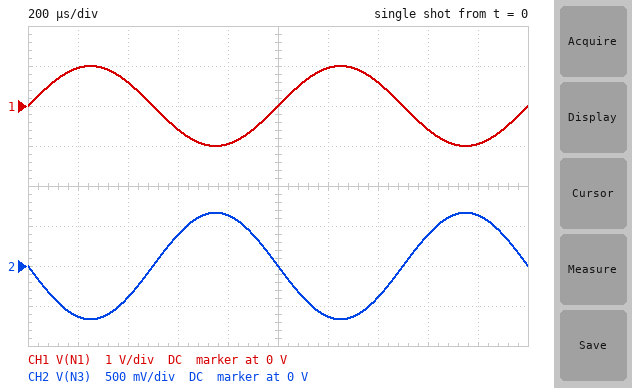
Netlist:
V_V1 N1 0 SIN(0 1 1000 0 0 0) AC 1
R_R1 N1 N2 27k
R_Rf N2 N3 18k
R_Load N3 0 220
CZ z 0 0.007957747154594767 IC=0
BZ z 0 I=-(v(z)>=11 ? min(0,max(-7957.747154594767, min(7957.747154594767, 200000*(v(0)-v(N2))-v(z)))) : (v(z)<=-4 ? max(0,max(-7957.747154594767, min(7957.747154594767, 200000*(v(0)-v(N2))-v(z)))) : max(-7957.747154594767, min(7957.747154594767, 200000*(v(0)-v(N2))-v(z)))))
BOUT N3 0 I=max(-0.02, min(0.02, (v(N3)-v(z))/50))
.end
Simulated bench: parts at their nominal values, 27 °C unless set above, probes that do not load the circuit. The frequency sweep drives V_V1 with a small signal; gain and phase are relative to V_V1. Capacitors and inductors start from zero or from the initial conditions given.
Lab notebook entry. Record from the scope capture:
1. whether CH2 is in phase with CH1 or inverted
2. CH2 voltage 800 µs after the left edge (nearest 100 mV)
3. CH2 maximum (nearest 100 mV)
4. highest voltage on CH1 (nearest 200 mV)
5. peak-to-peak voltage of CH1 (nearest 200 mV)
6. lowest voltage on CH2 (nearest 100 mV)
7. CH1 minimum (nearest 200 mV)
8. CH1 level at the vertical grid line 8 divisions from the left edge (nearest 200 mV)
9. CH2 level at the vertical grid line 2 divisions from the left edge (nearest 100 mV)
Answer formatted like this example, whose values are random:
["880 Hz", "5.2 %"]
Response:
["inverted", "600 mV", "700 mV", "1.0 V", "2.0 V", "-700 mV", "-1.0 V", "-600 mV", "-400 mV"]
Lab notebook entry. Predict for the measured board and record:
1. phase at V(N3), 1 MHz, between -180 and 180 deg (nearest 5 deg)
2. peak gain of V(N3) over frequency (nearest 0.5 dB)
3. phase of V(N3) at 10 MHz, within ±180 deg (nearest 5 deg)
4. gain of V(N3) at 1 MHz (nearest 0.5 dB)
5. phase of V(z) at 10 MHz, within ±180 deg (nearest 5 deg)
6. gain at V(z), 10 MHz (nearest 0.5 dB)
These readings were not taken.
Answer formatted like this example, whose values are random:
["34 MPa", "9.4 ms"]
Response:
["155 deg", "-3.5 dB", "100 deg", "-4.5 dB", "100 deg", "-16.0 dB"]
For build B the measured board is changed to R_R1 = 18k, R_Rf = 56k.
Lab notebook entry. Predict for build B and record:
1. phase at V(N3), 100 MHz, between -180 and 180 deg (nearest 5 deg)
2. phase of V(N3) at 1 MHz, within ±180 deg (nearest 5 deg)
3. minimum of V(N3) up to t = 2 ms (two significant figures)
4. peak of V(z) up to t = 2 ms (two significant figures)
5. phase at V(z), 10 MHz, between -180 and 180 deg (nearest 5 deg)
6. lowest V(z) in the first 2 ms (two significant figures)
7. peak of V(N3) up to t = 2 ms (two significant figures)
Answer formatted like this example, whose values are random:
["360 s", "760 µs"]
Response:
["90 deg", "130 deg", "-3.1 V", "3.8 V", "95 deg", "-3.8 V", "3.1 V"]
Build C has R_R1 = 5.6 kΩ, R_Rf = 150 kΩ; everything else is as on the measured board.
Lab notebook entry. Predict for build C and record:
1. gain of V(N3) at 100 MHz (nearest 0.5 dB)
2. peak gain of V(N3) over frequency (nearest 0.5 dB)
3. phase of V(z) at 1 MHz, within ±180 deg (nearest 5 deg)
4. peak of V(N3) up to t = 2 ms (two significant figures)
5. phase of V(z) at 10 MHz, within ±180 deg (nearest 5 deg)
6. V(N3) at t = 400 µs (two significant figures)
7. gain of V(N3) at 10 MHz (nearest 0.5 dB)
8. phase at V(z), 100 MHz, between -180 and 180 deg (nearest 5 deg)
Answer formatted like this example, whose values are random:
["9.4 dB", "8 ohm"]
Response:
["-30.0 dB", "28.5 dB", "95 deg", "4.4 V", "90 deg", "-3.3 V", "-10.0 dB", "90 deg"]
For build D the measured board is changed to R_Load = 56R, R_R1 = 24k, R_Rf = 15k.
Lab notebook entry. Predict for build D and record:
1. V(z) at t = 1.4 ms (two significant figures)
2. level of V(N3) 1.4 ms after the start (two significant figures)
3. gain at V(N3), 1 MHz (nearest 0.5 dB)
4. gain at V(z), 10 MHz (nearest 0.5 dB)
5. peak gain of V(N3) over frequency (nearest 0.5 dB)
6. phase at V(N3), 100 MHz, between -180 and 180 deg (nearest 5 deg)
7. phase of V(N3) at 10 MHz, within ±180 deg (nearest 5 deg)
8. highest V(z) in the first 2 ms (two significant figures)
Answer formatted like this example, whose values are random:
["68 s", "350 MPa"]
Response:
["-700 mV", "-370 mV", "-6.0 dB", "-16.5 dB", "-4.0 dB", "85 deg", "95 deg", "1.2 V"]
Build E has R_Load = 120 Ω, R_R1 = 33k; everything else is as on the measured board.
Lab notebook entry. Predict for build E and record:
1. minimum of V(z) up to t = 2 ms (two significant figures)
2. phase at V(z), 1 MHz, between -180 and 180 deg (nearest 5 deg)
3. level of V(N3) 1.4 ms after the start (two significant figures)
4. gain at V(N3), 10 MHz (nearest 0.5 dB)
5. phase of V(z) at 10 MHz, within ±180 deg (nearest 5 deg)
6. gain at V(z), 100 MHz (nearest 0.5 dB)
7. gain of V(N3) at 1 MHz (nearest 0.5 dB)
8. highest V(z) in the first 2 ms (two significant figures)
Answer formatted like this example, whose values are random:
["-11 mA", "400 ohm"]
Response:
["-770 mV", "150 deg", "-320 mV", "-20.0 dB", "100 deg", "-37.0 dB", "-6.5 dB", "770 mV"]
